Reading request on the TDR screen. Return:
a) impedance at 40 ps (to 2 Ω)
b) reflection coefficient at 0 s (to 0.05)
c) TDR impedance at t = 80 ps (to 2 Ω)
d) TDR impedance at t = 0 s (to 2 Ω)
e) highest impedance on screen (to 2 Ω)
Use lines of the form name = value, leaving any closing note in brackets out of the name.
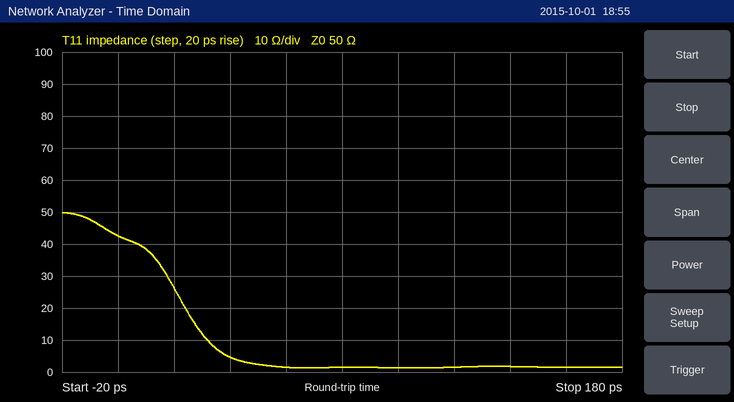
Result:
impedance at 40 ps = 4 Ω
reflection coefficient at 0 s = -0.10
TDR impedance at t = 80 ps = 2 Ω
TDR impedance at t = 0 s = 42 Ω
highest impedance on screen = 50 Ω
